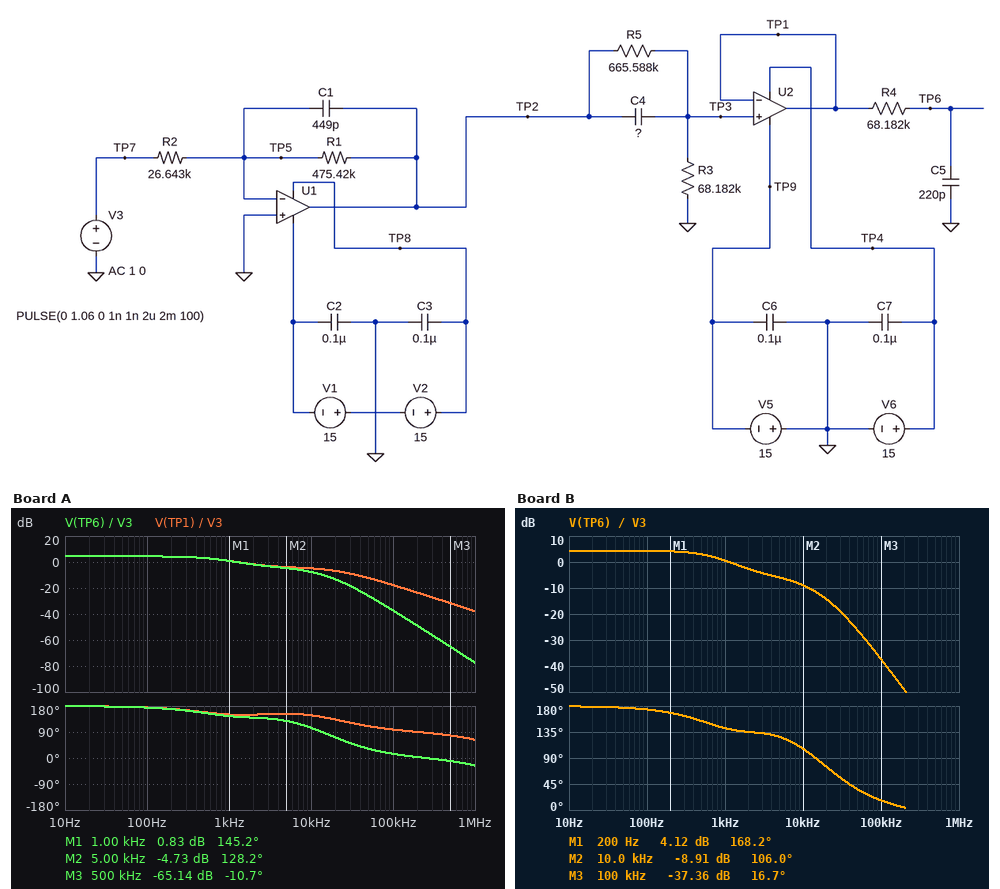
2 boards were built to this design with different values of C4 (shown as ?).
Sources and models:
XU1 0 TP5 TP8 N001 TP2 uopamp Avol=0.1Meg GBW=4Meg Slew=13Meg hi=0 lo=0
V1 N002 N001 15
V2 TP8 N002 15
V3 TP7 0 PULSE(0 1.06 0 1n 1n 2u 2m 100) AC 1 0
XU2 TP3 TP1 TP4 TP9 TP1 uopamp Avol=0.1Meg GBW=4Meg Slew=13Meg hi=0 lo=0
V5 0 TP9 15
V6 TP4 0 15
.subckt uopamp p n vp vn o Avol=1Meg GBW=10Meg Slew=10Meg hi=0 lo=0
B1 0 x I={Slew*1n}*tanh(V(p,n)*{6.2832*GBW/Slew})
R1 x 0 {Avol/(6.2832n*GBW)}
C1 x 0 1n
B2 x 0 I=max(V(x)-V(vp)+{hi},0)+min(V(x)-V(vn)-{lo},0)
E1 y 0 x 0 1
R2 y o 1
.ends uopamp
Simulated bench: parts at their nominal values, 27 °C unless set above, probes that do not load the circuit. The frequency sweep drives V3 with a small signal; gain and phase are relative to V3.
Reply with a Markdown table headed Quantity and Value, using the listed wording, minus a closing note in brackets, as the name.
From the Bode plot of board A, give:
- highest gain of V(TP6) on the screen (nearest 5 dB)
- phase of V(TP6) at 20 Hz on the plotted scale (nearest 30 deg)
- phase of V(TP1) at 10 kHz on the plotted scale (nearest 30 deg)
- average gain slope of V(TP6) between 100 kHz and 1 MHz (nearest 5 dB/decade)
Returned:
| Quantity | Value |
|---|---|
| highest gain of V(TP6) on the screen | 5 dB |
| phase of V(TP6) at 20 Hz on the plotted scale | 180 deg |
| phase of V(TP1) at 10 kHz on the plotted scale | 150 deg |
| average gain slope of V(TP6) between 100 kHz and 1 MHz | -40 dB/decade |
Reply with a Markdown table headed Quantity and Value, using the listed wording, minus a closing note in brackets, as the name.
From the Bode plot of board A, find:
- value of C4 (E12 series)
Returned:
| Quantity | Value |
|---|---|
| value of C4 | 120 pF |
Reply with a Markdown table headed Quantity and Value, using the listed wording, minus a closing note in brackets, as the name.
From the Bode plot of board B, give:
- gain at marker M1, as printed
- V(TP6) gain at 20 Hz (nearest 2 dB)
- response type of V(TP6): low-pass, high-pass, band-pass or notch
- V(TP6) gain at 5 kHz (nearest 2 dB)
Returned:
| Quantity | Value |
|---|---|
| gain at marker M1, as printed | 4.12 dB |
| V(TP6) gain at 20 Hz | 4 dB |
| response type of V(TP6): low-pass, high-pass, band-pass or notch | low-pass |
| V(TP6) gain at 5 kHz | -6 dB |
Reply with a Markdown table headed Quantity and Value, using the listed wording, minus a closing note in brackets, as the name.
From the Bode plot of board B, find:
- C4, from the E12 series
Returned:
| Quantity | Value |
|---|---|
| C4, from the E12 series | 100 pF |
